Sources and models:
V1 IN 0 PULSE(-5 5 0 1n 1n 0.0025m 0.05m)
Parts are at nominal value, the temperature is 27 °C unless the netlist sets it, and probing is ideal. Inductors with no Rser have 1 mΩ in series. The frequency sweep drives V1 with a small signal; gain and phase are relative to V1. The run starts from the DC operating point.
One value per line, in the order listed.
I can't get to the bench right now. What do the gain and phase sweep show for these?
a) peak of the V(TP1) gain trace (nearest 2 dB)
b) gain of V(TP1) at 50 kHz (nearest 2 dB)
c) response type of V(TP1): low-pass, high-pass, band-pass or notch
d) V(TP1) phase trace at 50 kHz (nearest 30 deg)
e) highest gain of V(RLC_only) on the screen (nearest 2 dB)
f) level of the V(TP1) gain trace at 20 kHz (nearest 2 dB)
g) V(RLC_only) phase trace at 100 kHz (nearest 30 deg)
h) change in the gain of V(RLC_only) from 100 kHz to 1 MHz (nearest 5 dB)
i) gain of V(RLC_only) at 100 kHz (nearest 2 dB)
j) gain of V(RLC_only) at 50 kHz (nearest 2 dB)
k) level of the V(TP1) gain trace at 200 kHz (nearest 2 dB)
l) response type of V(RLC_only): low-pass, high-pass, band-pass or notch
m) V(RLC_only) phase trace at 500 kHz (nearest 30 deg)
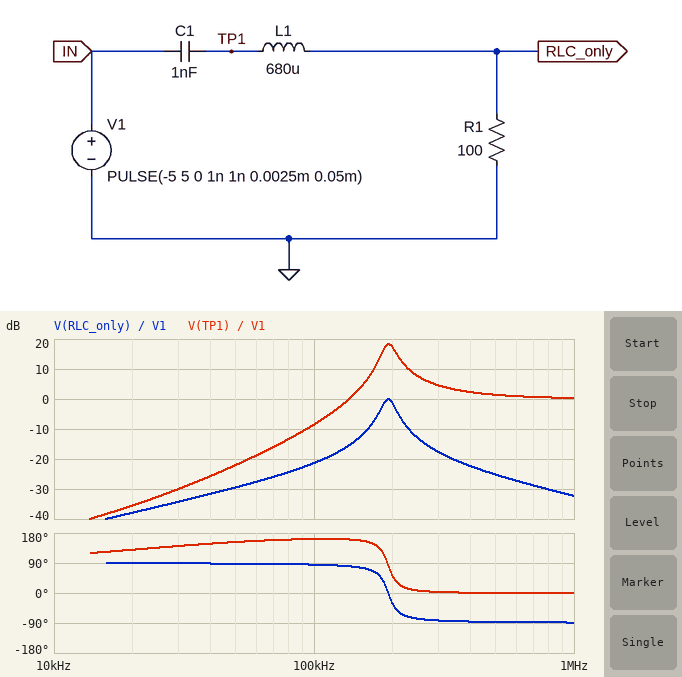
18 dB
-22 dB
high-pass
150 deg
0 dB
-36 dB
90 deg
-10 dB
-22 dB
-30 dB
18 dB
band-pass
-90 deg
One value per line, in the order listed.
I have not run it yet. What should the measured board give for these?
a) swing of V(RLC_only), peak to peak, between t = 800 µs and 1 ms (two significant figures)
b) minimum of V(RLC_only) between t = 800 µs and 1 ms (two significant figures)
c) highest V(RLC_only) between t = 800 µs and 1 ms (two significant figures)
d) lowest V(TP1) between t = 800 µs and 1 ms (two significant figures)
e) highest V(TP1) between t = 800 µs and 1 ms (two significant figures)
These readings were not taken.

3.6 V
-2.0 V
1.6 V
-18 V
15 V
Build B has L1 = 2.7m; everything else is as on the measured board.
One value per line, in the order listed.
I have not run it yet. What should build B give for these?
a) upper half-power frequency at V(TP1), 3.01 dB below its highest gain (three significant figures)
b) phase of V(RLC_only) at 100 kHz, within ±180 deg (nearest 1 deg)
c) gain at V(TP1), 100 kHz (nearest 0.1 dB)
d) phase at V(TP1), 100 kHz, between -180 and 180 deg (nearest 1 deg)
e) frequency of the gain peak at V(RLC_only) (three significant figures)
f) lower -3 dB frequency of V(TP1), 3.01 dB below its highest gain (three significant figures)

100 kHz
-46 deg
21.4 dB
40 deg
96.9 kHz
94.1 kHz
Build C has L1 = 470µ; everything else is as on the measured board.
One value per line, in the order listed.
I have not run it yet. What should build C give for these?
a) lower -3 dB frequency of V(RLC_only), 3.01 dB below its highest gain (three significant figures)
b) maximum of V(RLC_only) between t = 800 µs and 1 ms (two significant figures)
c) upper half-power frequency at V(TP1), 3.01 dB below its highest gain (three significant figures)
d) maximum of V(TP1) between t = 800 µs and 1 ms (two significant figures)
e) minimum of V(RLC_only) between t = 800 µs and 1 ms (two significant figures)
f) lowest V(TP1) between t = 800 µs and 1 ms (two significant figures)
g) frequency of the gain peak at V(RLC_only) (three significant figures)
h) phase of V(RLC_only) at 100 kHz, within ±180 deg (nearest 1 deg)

216 kHz
1.8 V
253 kHz
14 V
-2.3 V
-17 V
232 kHz
86 deg
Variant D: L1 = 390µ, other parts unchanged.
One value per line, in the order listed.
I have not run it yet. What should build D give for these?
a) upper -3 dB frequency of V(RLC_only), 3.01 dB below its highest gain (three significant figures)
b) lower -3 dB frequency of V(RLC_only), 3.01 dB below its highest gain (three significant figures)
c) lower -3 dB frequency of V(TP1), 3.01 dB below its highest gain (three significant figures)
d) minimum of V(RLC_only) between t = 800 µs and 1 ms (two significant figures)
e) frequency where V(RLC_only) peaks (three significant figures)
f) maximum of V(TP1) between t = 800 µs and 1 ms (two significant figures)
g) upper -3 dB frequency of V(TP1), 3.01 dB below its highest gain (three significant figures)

276 kHz
235 kHz
238 kHz
-2.3 V
255 kHz
13 V
280 kHz
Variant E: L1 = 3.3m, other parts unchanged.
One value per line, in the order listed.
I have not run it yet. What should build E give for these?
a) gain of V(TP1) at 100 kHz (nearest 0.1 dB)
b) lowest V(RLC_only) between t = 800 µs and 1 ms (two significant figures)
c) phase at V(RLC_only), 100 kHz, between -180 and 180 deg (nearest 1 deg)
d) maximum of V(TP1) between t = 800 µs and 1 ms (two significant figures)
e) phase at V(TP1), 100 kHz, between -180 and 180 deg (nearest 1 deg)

12.5 dB
-470 mV
-78 deg
8.2 V
9 deg
